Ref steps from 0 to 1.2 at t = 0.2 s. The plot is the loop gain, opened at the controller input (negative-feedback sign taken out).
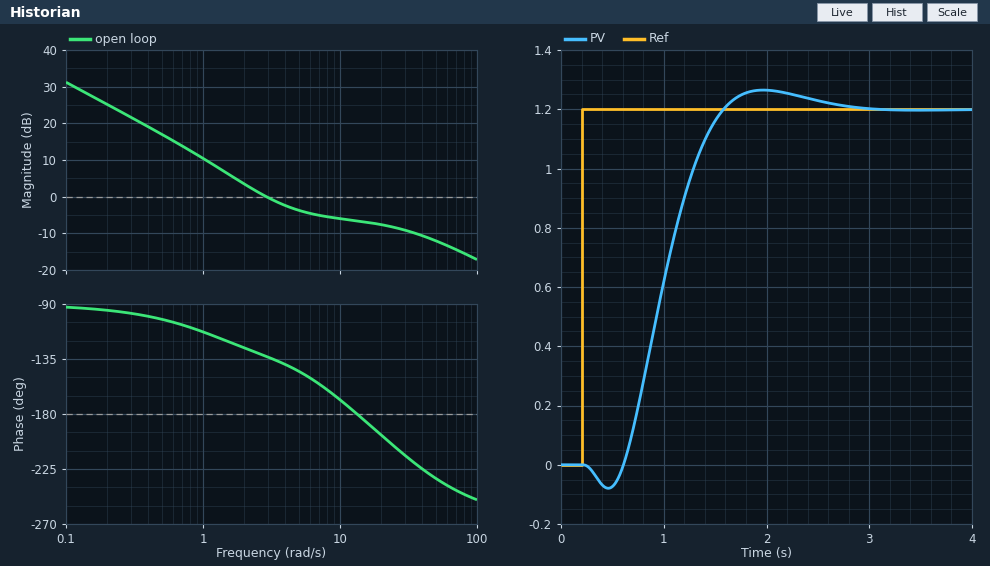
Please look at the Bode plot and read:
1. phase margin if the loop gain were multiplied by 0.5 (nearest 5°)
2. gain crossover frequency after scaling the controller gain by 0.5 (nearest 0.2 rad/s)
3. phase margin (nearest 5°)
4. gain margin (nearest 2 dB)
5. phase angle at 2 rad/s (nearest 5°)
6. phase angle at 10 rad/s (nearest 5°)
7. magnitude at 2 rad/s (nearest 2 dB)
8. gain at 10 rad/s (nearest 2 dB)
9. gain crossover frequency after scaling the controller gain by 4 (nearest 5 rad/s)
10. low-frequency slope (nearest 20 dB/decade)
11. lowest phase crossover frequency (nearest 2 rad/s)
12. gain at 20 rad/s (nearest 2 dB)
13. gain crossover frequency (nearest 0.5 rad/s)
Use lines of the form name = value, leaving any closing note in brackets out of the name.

phase margin if the loop gain were multiplied by 0.5 = 60°
gain crossover frequency after scaling the controller gain by 0.5 = 1.6 rad/s
phase margin = 45°
gain margin = 6 dB
phase angle at 2 rad/s = -125°
phase angle at 10 rad/s = -170°
magnitude at 2 rad/s = 4 dB
gain at 10 rad/s = -6 dB
gain crossover frequency after scaling the controller gain by 4 = 50 rad/s
low-frequency slope = -20 dB/decade
lowest phase crossover frequency = 14 rad/s
gain at 20 rad/s = -8 dB
gain crossover frequency = 3.0 rad/s
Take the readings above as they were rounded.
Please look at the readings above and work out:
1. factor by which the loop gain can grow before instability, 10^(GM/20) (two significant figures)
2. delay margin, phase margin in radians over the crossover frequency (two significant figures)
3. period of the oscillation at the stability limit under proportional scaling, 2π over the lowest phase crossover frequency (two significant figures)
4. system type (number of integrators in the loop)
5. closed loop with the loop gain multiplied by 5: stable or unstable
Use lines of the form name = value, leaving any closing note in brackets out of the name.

factor by which the loop gain can grow before instability, 10^(GM/20) = 2.0
delay margin, phase margin in radians over the crossover frequency = 0.26 s
period of the oscillation at the stability limit under proportional scaling, 2π over the lowest phase crossover frequency = 0.45 s
system type = 1
closed loop with the loop gain multiplied by 5: stable or unstable = unstable
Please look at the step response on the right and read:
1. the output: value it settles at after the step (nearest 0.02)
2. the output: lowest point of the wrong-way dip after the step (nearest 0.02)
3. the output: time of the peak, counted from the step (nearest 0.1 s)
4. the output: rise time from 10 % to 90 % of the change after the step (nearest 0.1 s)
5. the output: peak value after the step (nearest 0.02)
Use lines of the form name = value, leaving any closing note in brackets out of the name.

the output: value it settles at after the step = 1.20
the output: lowest point of the wrong-way dip after the step = -0.08
the output: time of the peak, counted from the step = 1.8 s
the output: rise time from 10 % to 90 % of the change after the step = 0.7 s
the output: peak value after the step = 1.26
